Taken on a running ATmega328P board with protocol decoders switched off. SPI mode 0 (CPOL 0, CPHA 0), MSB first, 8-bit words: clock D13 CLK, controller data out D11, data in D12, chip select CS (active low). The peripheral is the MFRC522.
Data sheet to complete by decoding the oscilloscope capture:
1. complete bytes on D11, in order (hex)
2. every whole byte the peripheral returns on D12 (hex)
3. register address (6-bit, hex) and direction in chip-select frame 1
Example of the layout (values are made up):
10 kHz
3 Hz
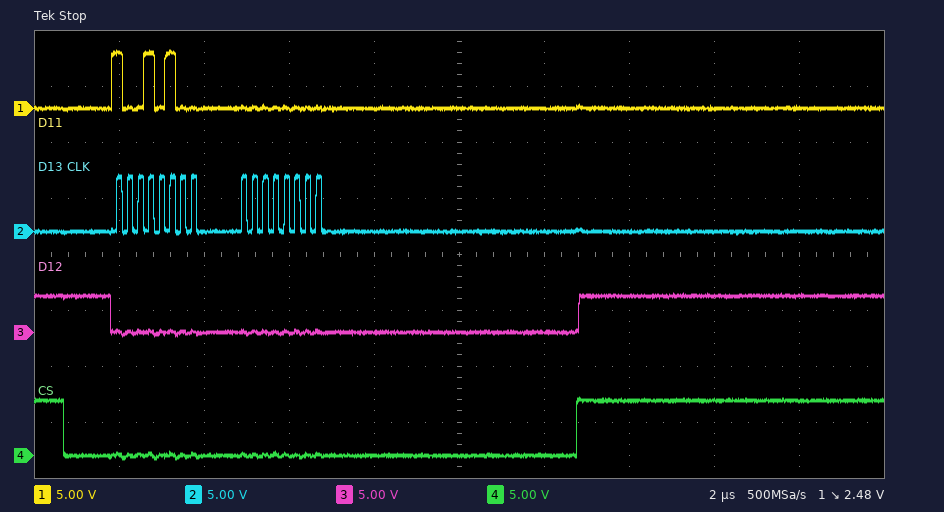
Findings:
0x94 0x00
0x00 0x00
0x0A read
